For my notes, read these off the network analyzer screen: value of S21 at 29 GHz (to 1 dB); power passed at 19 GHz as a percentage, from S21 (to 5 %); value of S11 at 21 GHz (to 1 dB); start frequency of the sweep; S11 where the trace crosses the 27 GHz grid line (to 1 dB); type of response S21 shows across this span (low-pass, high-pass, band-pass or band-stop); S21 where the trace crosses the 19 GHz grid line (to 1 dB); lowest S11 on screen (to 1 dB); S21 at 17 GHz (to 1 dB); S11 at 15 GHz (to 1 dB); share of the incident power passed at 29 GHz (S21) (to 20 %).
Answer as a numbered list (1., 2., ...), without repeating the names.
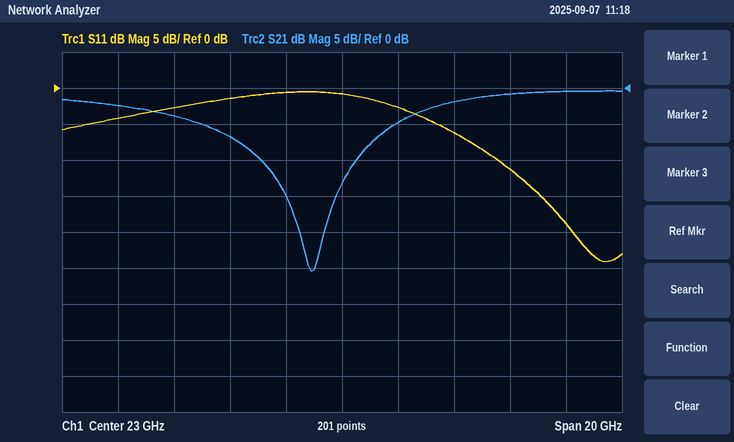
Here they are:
1. -1 dB
2. 20 %
3. -1 dB
4. 13 GHz
5. -6 dB
6. band-stop
7. -7 dB
8. -24 dB
9. -4 dB
10. -4 dB
11. 80 %
